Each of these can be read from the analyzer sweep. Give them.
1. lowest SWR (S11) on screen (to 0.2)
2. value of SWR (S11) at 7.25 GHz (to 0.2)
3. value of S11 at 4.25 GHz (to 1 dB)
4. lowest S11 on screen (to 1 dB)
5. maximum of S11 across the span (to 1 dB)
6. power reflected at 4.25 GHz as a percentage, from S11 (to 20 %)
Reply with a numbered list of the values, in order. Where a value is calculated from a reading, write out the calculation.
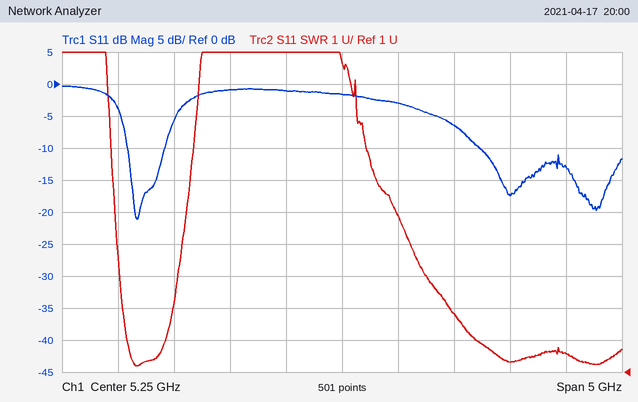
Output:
1. 1.2
2. 1.6
3. -1 dB
4. -21 dB
5. 0 dB
6. 10^(-1/10) ≈ 79.4 %, so 80 % to the nearest 20 %
